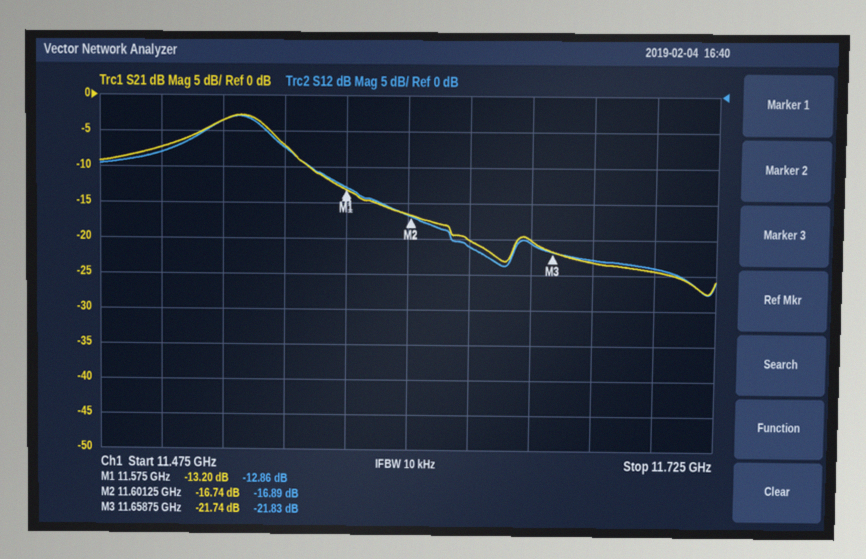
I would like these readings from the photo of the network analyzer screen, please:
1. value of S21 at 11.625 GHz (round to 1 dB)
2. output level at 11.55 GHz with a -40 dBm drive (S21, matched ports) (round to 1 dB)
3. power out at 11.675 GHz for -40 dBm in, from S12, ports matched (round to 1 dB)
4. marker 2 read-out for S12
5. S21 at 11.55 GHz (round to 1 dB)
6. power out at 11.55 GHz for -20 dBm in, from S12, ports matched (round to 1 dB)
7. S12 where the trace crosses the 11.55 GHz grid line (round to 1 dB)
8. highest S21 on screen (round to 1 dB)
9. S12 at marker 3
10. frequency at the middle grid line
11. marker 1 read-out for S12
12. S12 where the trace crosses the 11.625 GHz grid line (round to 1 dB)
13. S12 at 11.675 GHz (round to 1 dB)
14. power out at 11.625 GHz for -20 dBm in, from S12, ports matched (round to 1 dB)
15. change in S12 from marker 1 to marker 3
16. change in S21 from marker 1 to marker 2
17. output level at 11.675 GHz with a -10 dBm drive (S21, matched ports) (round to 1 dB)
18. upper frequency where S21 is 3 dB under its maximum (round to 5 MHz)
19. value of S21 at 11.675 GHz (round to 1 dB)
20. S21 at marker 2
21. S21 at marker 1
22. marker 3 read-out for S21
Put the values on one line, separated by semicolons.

-20 dB; -47 dBm; -63 dBm; -16.89 dB; -7 dB; -27 dBm; -7 dB; -3 dB; -21.83 dB; 11.6 GHz; -12.86 dB; -21 dB; -23 dB; -41 dBm; -8.97 dB; -3.54 dB; -33 dBm; 11.545 GHz; -23 dB; -16.74 dB; -13.20 dB; -21.74 dB
